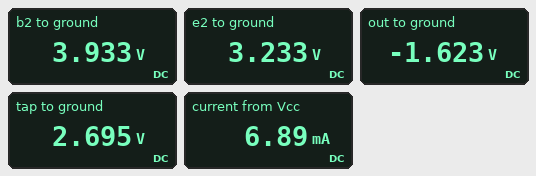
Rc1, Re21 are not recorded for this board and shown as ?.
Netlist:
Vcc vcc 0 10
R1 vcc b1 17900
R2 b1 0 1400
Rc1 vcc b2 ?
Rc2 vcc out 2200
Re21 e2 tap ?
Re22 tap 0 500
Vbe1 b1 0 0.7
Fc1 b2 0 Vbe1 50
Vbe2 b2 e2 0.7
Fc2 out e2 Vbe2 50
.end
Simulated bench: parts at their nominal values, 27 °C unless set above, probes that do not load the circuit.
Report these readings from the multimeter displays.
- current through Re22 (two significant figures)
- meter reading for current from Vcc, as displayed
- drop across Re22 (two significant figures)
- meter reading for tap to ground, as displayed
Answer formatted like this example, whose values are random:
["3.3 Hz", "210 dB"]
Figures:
["5.4 mA", "6.89 mA", "2.7 V", "2.695 V"]
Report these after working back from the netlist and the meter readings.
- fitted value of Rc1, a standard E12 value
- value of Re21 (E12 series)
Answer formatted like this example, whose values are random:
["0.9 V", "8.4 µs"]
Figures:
["5.6 kΩ", "100 Ω"]
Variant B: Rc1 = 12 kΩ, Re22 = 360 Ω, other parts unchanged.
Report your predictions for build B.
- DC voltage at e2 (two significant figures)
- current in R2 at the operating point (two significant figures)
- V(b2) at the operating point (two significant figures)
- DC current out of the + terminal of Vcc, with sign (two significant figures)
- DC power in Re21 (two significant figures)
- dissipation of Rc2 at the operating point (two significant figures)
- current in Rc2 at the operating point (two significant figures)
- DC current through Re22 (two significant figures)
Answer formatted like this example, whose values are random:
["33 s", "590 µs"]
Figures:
["-1.6 V", "500 µA", "-910 mV", "-2.0 mA", "1.2 mW", "26 mW", "3.4 mA", "3.5 mA"]
